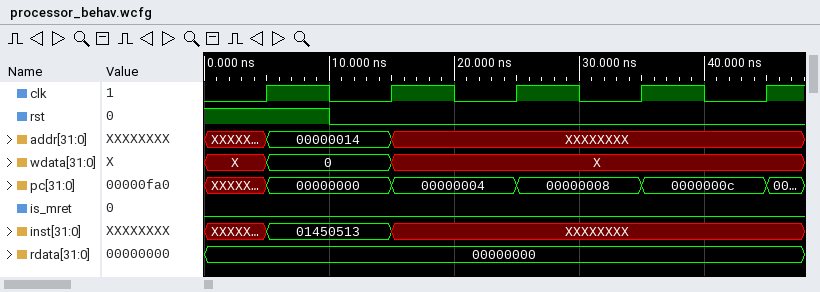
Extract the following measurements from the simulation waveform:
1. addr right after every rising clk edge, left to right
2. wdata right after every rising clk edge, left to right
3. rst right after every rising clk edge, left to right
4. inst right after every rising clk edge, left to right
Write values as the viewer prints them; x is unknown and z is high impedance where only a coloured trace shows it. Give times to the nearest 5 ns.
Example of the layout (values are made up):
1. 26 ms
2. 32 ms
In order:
1. 00000014, XXXXXXXX, XXXXXXXX, XXXXXXXX, XXXXXXXX
2. 0, X, X, X, X
3. 1 0 0 0 0
4. 01450513, XXXXXXXX, XXXXXXXX, XXXXXXXX, XXXXXXXX
